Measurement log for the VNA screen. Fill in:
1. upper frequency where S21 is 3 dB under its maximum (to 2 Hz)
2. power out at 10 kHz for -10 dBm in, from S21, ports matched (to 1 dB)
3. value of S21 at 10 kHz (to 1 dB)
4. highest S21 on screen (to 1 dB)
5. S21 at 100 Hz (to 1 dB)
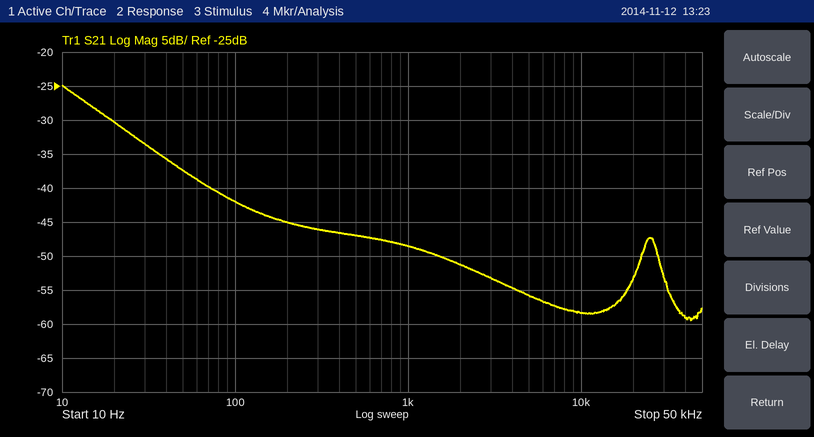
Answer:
14 Hz
-68 dBm
-58 dB
-25 dB
-42 dB
